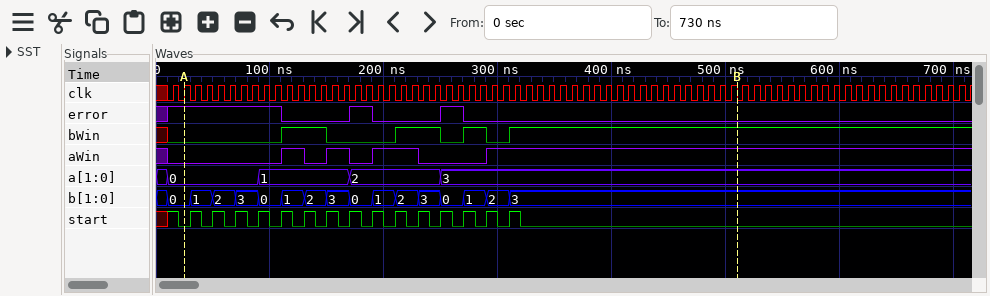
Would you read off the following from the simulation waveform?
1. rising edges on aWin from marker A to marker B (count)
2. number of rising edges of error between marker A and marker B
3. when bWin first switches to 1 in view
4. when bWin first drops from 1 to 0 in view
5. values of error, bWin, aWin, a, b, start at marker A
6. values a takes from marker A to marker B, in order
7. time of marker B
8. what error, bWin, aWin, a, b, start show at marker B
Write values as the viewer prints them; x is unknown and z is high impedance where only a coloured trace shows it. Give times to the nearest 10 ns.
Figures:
4
2
110 ns
150 ns
error=1, bWin=0, aWin=0, a=0, b=0, start=0
0, 1, 2, 3
510 ns
error=0, bWin=1, aWin=1, a=3, b=3, start=0
